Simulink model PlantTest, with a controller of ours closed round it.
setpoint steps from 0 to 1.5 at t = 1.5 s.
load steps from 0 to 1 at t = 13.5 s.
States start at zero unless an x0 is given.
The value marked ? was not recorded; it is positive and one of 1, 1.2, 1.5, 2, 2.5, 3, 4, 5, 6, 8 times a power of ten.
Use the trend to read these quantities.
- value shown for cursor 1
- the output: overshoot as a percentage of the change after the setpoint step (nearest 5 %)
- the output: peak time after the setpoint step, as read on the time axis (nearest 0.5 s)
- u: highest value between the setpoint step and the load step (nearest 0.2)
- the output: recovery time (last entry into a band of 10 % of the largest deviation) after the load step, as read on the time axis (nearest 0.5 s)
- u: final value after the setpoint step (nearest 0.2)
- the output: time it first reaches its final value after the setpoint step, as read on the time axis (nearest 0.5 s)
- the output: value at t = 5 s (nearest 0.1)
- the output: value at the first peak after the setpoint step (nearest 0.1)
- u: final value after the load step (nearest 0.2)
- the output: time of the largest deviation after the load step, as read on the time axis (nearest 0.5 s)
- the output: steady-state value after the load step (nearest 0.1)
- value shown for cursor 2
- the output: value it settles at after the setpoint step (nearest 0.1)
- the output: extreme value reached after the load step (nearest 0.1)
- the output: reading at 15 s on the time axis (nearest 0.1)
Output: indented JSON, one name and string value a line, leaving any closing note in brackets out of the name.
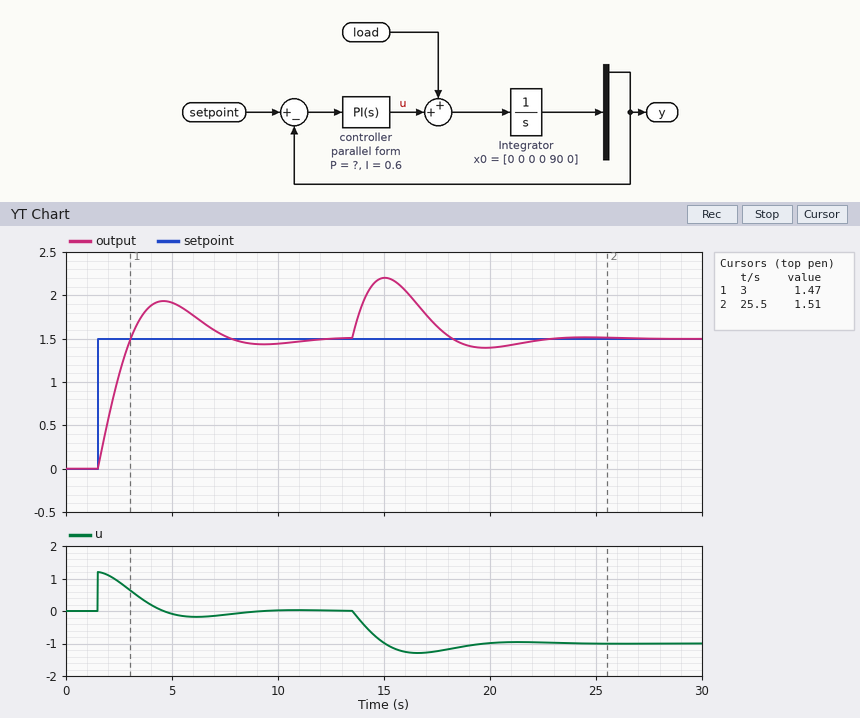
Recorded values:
{
  "value shown for cursor 1": "1.47",
  "the output: overshoot as a percentage of the change after the setpoint step": "30 %",
  "the output: peak time after the setpoint step, as read on the time axis": "4.5 s",
  "u: highest value between the setpoint step and the load step": "1.2",
  "the output: recovery time (last entry into a band of 10 % of the largest deviation) after the load step, as read on the time axis": "21.0 s",
  "u: final value after the setpoint step": "0.0",
  "the output: time it first reaches its final value after the setpoint step, as read on the time axis": "3.0 s",
  "the output: value at t = 5 s": "1.9",
  "the output: value at the first peak after the setpoint step": "1.9",
  "u: final value after the load step": "-1.0",
  "the output: time of the largest deviation after the load step, as read on the time axis": "15.0 s",
  "the output: steady-state value after the load step": "1.5",
  "value shown for cursor 2": "1.51",
  "the output: value it settles at after the setpoint step": "1.5",
  "the output: extreme value reached after the load step": "2.2",
  "the output: reading at 15 s on the time axis": "2.2"
}
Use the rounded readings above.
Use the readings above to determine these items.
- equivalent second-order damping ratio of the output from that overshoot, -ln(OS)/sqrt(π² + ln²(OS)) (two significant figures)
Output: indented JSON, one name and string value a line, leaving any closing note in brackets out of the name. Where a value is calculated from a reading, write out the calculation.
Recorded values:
{
  "equivalent second-order damping ratio of the output from that overshoot, -ln(OS)/sqrt(π² + ln²(OS))": "ln(0.3) = -1.204; 1.204 / sqrt(9.870 + 1.450) = 0.36"
}
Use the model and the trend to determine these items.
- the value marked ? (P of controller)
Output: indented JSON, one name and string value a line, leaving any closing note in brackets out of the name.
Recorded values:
{
  "the value marked ?": "0.8"
}
